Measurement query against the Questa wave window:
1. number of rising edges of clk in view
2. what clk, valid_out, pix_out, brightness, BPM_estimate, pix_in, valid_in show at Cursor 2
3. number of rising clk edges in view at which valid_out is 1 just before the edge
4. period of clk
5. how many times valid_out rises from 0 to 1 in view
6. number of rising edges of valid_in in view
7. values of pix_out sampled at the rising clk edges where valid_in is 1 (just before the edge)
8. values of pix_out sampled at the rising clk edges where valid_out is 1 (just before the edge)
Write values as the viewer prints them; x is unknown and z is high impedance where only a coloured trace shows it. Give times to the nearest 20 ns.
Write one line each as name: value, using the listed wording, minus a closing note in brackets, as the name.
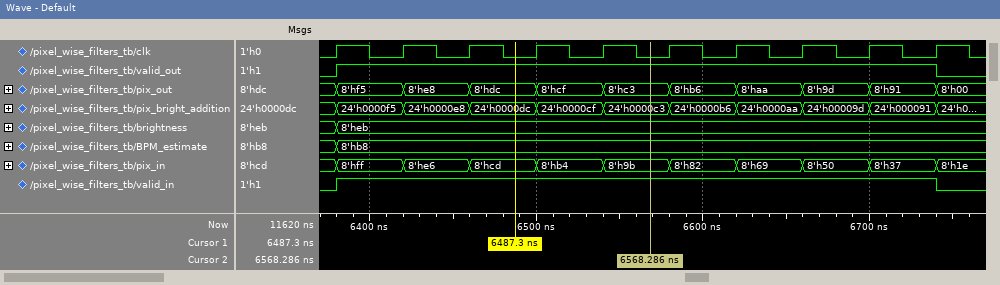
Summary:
number of rising edges of clk in view: 10
what clk, valid_out, pix_out, brightness, BPM_estimate, pix_in, valid_in show at Cursor 2: clk=0, valid_out=1, pix_out=8'hc3, brightness=8'heb, BPM_estimate=8'hb8, pix_in=8'h9b, valid_in=1
number of rising clk edges in view at which valid_out is 1 just before the edge: 9
period of clk: 40 ns
how many times valid_out rises from 0 to 1 in view: 1
number of rising edges of valid_in in view: 1
values of pix_out sampled at the rising clk edges where valid_in is 1: 8'hf5, 8'he8, 8'hdc, 8'hcf, 8'hc3, 8'hb6, 8'haa, 8'h9d, 8'h91
values of pix_out sampled at the rising clk edges where valid_out is 1: 8'hf5, 8'he8, 8'hdc, 8'hcf, 8'hc3, 8'hb6, 8'haa, 8'h9d, 8'h91
